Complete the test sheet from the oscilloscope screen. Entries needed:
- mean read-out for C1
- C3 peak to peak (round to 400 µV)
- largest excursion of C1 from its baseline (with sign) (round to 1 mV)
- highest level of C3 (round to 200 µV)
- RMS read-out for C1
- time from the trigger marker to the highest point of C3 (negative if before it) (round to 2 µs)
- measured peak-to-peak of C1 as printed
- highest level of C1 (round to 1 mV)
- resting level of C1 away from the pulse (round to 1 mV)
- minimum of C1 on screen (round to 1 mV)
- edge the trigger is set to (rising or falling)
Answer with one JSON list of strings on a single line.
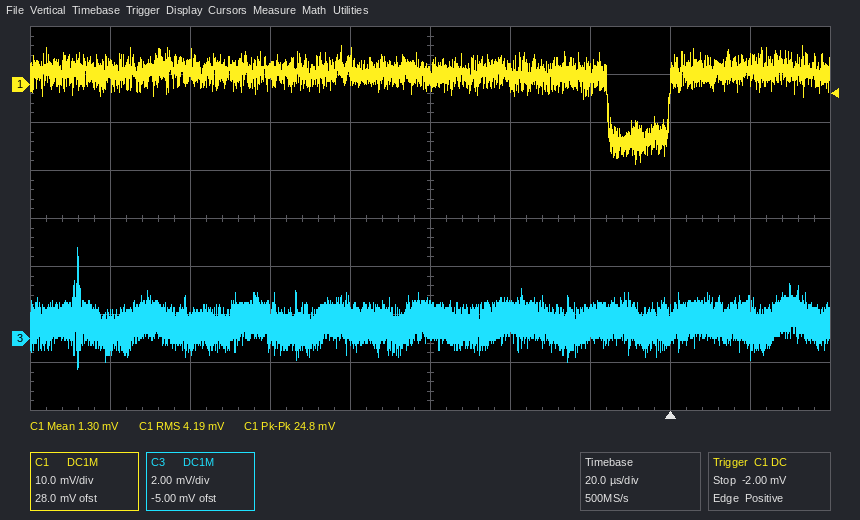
["1.30 mV", "5.2 mV", "-19 mV", "3.8 mV", "4.19 mV", "-148 µs", "24.8 mV", "8 mV", "2 mV", "-17 mV", "rising"]
